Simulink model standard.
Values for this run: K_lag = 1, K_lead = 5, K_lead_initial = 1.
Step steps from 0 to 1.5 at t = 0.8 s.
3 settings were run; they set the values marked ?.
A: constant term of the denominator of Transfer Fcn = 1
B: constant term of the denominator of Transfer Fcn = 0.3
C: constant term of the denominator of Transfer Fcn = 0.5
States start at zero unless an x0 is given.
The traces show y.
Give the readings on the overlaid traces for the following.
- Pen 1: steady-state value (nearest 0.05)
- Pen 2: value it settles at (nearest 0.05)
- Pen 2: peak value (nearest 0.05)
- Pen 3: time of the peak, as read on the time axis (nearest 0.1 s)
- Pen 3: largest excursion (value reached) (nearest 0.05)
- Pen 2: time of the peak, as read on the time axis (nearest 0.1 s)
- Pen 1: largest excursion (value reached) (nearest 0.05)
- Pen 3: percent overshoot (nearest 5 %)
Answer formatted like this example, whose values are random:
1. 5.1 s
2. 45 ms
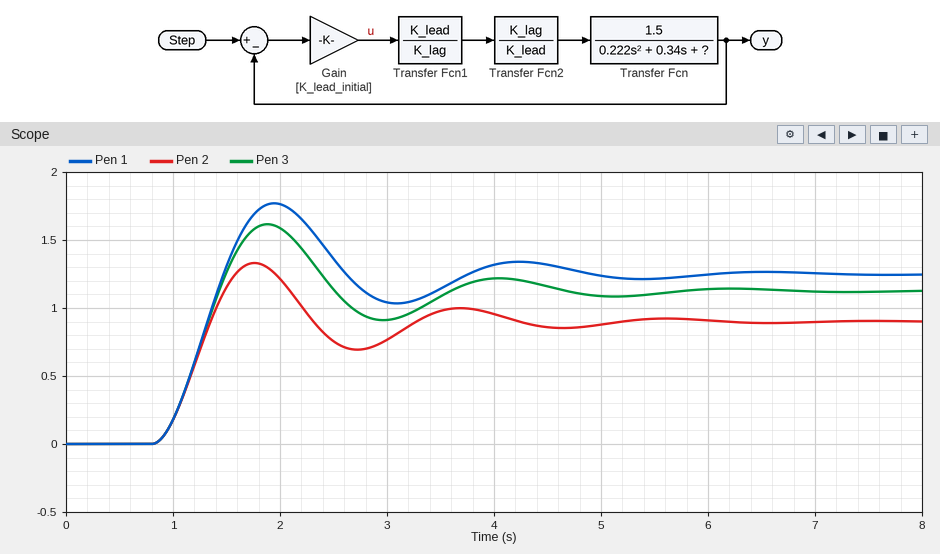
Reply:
1. 1.25
2. 0.90
3. 1.35
4. 1.9 s
5. 1.60
6. 1.8 s
7. 1.75
8. 45 %
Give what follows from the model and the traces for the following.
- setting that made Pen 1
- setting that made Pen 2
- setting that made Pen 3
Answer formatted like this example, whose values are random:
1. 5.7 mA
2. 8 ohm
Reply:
1. B
2. A
3. C
